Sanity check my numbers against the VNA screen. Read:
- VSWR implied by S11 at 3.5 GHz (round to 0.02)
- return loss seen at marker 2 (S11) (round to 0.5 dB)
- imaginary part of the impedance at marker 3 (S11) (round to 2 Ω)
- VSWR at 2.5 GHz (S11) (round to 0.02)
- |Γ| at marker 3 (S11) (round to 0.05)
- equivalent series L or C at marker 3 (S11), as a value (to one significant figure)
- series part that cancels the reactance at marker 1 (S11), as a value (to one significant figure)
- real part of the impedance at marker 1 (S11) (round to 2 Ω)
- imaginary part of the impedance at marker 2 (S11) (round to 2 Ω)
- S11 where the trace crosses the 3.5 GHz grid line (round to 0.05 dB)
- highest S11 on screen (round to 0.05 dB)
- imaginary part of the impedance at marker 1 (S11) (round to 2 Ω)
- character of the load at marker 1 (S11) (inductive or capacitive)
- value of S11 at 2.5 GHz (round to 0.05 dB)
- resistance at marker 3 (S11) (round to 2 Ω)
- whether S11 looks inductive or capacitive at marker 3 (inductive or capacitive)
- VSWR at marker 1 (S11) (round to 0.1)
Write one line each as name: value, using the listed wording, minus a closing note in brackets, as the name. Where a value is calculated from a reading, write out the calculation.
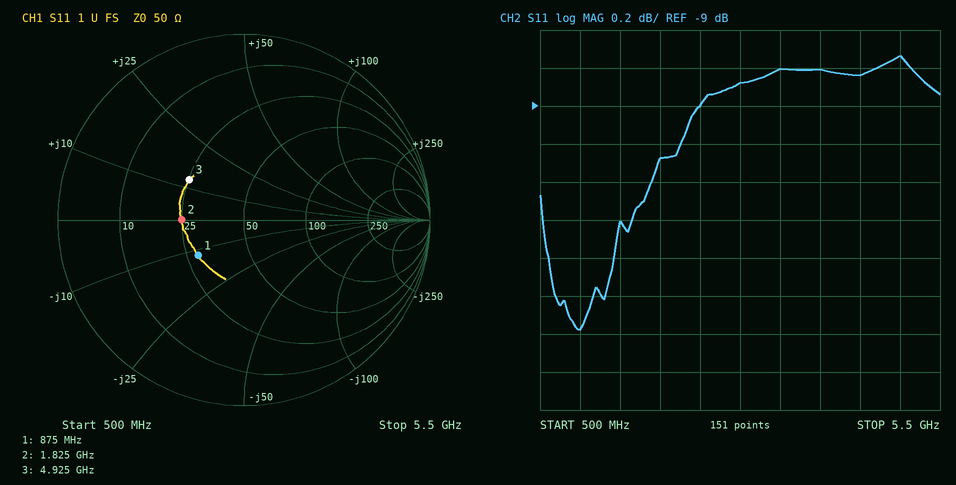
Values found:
VSWR implied by S11 at 3.5 GHz: |Γ| = 10^(-8.8/20) = 0.3631; VSWR = (1 + 0.3631)/(1 − 0.3631) ≈ 2.14
return loss seen at marker 2 (S11): 9.5 dB
imaginary part of the impedance at marker 3 (S11): +12 Ω
VSWR at 2.5 GHz (S11): |Γ| = 10^(-9/20) = 0.3548; VSWR = (1 + 0.3548)/(1 − 0.3548) ≈ 2.10
|Γ| at marker 3 (S11): 0.35
equivalent series L or C at marker 3 (S11), as a value: L = 12 Ω/(2π × 4.925 GHz) ≈ 388 pH, so 400 pH to one significant figure
series part that cancels the reactance at marker 1 (S11), as a value: L = 12 Ω/(2π × 875 MHz) ≈ 2 nH
real part of the impedance at marker 1 (S11): 28 Ω
imaginary part of the impedance at marker 2 (S11): 0 Ω
S11 where the trace crosses the 3.5 GHz grid line: -8.80 dB
highest S11 on screen: -8.75 dB
imaginary part of the impedance at marker 1 (S11): -12 Ω
character of the load at marker 1 (S11): capacitive
value of S11 at 2.5 GHz: -9.00 dB
resistance at marker 3 (S11): 26 Ω
whether S11 looks inductive or capacitive at marker 3: inductive
VSWR at marker 1 (S11): 1.9
